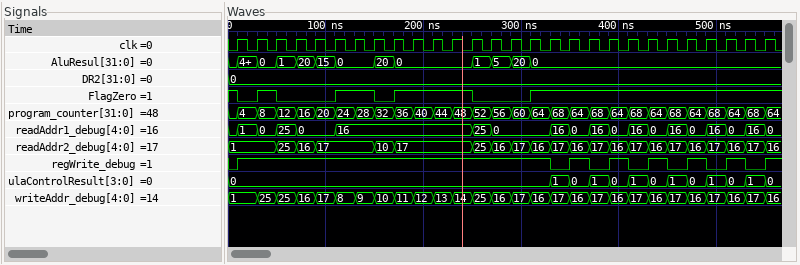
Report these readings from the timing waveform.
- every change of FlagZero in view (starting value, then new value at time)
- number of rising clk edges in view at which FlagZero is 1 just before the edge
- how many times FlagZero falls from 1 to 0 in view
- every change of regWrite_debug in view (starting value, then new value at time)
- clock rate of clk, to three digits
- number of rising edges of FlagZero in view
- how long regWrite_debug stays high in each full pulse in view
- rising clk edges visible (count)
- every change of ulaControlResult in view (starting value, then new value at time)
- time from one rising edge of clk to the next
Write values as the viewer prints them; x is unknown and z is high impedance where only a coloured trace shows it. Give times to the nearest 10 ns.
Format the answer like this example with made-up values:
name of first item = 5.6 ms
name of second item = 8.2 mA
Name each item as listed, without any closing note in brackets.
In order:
every change of FlagZero in view = 1, 0 at 10 ns, 1 at 30 ns, 0 at 50 ns, 1 at 110 ns, 0 at 150 ns, 1 at 170 ns, 0 at 250 ns, 1 at 310 ns
number of rising clk edges in view at which FlagZero is 1 just before the edge = 20
how many times FlagZero falls from 1 to 0 in view = 4
every change of regWrite_debug in view = 0, 1 at 10 ns, 0 at 330 ns, 1 at 350 ns, 0 at 370 ns, 1 at 390 ns, 0 at 410 ns, 1 at 430 ns, 0 at 450 ns, 1 at 470 ns, 0 at 490 ns, 1 at 510 ns, 0 at 530 ns, 1 at 550 ns
clock rate of clk, to three digits = 50.0 MHz
number of rising edges of FlagZero in view = 4
how long regWrite_debug stays high in each full pulse in view = 320 ns, 20 ns, 20 ns, 20 ns, 20 ns, 20 ns
rising clk edges visible = 28
every change of ulaControlResult in view = 0, 1 at 330 ns, 0 at 350 ns, 1 at 370 ns, 0 at 390 ns, 1 at 410 ns, 0 at 430 ns, 1 at 450 ns, 0 at 470 ns, 1 at 490 ns, 0 at 510 ns, 1 at 530 ns, 0 at 550 ns
time from one rising edge of clk to the next = 20 ns
